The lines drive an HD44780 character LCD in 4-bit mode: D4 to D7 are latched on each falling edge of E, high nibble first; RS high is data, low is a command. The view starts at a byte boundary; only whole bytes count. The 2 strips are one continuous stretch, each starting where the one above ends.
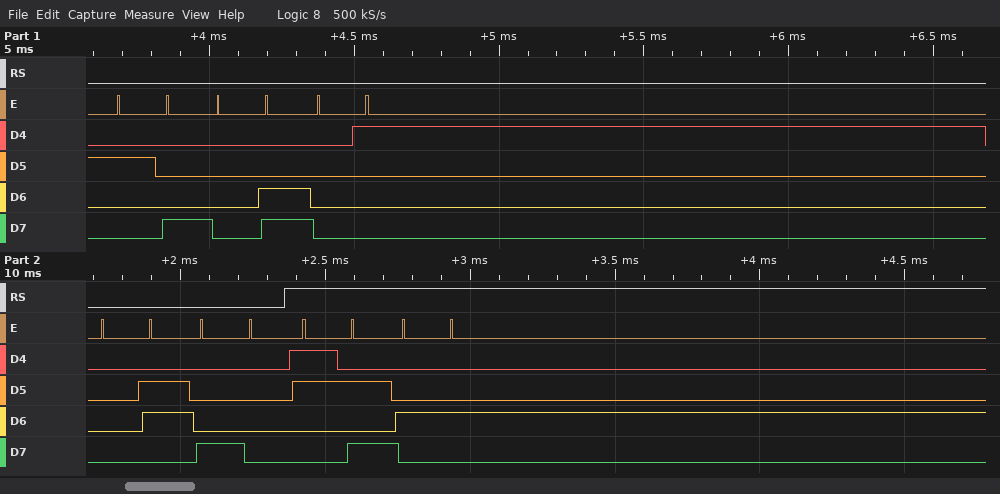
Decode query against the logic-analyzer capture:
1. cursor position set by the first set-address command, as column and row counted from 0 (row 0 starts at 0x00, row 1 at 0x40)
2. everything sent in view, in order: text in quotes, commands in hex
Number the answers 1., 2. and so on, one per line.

1. column 0, row 0
2. 0x28 0x0C 0x01 0x06 0x80 ":D"
